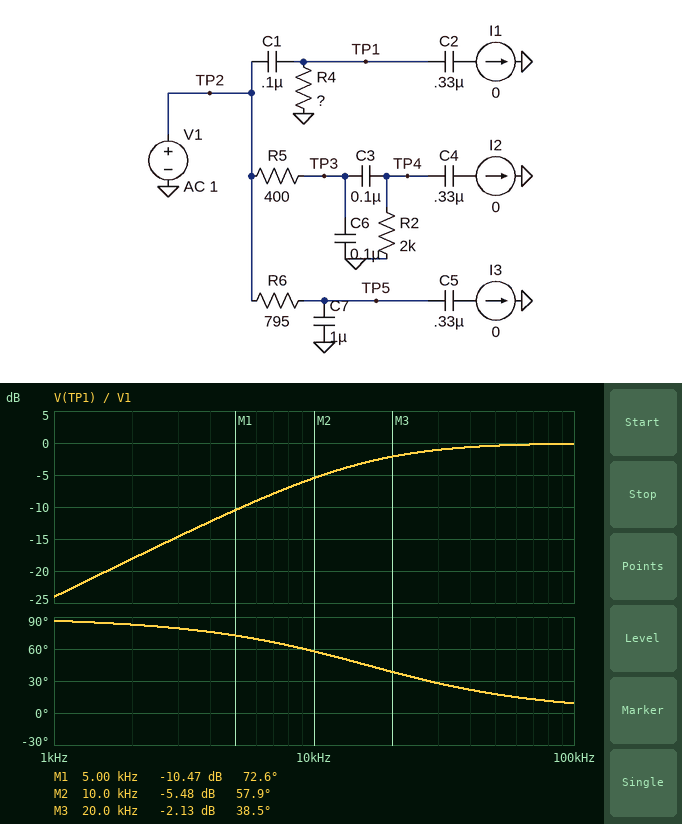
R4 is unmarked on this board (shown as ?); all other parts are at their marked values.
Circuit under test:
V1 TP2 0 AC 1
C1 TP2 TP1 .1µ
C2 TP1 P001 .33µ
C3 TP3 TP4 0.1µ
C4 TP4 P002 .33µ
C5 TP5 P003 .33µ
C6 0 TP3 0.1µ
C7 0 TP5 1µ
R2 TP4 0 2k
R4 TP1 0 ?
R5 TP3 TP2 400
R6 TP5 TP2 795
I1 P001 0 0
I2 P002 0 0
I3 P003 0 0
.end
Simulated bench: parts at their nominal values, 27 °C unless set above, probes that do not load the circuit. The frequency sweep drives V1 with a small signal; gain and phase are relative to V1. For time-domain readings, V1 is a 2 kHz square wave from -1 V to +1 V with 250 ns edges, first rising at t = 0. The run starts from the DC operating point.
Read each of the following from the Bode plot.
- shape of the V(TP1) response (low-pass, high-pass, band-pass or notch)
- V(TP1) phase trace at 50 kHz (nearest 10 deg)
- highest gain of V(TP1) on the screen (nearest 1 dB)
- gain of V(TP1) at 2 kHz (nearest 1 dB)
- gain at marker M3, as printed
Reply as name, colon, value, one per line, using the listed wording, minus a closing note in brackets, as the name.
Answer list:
shape of the V(TP1) response: high-pass
V(TP1) phase trace at 50 kHz: 20 deg
highest gain of V(TP1) on the screen: 0 dB
gain of V(TP1) at 2 kHz: -18 dB
gain at marker M3, as printed: -2.13 dB
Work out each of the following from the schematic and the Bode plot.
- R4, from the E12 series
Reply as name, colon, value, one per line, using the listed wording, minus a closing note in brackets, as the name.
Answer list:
R4, from the E12 series: 100 Ω
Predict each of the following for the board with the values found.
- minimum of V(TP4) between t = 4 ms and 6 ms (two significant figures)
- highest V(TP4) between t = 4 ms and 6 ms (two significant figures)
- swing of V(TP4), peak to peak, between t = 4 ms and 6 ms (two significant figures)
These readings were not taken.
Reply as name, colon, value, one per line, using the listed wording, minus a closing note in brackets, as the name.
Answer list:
minimum of V(TP4) between t = 4 ms and 6 ms: -830 mV
highest V(TP4) between t = 4 ms and 6 ms: 830 mV
swing of V(TP4), peak to peak, between t = 4 ms and 6 ms: 1.7 V
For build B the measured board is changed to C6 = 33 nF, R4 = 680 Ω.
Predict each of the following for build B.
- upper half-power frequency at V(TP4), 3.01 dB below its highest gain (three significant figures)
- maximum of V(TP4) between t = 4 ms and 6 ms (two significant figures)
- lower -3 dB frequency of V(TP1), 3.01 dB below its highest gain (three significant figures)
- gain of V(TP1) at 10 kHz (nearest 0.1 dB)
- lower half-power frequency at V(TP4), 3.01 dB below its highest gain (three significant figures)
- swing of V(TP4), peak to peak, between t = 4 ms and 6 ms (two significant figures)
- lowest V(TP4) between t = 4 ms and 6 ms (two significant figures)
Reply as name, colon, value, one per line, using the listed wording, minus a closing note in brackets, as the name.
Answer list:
upper half-power frequency at V(TP4), 3.01 dB below its highest gain: 15.9 kHz
maximum of V(TP4) between t = 4 ms and 6 ms: 1.0 V
lower -3 dB frequency of V(TP1), 3.01 dB below its highest gain: 2.34 kHz
gain of V(TP1) at 10 kHz: -0.2 dB
lower half-power frequency at V(TP4), 3.01 dB below its highest gain: 605 Hz
swing of V(TP4), peak to peak, between t = 4 ms and 6 ms: 2.1 V
lowest V(TP4) between t = 4 ms and 6 ms: -1.0 V
